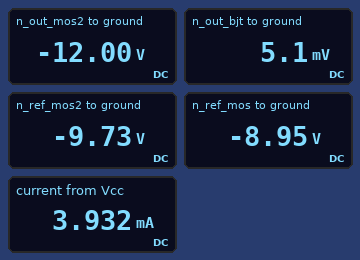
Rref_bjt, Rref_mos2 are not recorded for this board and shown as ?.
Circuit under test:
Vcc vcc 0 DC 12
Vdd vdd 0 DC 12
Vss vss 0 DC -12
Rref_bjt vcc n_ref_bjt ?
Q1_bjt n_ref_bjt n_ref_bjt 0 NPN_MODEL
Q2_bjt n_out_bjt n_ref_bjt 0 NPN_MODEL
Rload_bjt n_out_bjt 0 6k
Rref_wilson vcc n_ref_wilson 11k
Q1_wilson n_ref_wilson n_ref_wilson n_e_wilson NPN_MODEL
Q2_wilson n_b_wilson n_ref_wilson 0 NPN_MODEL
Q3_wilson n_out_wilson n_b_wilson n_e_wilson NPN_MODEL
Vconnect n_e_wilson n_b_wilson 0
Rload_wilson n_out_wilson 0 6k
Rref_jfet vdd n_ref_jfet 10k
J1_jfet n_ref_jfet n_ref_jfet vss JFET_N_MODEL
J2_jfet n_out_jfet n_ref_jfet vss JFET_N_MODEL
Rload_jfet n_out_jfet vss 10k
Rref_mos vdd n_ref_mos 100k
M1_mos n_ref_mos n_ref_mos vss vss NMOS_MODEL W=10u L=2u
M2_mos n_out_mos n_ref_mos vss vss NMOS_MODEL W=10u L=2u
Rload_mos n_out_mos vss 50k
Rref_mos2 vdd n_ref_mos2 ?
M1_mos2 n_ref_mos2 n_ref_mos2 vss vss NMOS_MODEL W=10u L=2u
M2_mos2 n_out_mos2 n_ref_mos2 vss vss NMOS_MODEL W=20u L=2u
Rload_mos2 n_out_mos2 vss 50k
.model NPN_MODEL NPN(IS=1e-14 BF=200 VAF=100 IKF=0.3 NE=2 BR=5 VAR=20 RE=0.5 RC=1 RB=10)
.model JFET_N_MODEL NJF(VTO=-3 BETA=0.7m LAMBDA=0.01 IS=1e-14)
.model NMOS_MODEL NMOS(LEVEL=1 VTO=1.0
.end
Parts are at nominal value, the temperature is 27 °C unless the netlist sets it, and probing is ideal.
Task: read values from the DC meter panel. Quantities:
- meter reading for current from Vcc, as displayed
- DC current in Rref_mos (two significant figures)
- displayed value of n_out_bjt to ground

3.932 mA
210 µA
5.1 mV
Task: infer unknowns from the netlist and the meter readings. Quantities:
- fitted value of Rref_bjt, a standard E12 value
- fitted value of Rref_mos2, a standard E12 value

3.9 kΩ
270 kΩ
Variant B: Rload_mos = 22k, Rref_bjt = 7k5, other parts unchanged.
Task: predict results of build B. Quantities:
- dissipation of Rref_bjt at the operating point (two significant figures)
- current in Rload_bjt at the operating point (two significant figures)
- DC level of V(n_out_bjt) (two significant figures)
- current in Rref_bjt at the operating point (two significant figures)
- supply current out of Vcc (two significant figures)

17 mW
830 nA
5.0 mV
1.5 mA
2.5 mA
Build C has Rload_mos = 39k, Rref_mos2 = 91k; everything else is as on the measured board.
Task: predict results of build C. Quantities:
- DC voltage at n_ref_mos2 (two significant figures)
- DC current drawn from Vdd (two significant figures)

-8.9 V
2.8 mA
